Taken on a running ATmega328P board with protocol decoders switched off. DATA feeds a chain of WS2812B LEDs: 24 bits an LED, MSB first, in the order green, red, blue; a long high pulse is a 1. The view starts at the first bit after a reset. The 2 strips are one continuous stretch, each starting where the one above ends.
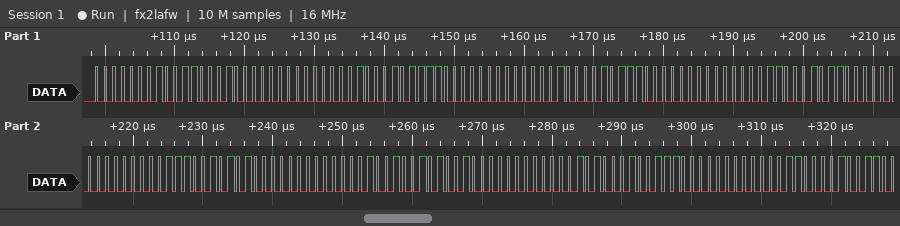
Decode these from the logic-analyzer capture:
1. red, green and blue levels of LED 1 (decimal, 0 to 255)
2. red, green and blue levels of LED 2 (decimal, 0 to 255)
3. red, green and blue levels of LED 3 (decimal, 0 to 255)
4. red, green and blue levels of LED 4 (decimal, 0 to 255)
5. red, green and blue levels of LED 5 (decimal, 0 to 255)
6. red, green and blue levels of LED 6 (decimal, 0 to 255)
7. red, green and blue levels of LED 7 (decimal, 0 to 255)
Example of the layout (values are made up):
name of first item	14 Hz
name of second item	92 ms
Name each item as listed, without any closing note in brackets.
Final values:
red, green and blue levels of LED 1	49, 1, 0
red, green and blue levels of LED 2	47, 2, 0
red, green and blue levels of LED 3	46, 4, 0
red, green and blue levels of LED 4	44, 6, 0
red, green and blue levels of LED 5	42, 7, 0
red, green and blue levels of LED 6	41, 9, 0
red, green and blue levels of LED 7	39, 10, 0
